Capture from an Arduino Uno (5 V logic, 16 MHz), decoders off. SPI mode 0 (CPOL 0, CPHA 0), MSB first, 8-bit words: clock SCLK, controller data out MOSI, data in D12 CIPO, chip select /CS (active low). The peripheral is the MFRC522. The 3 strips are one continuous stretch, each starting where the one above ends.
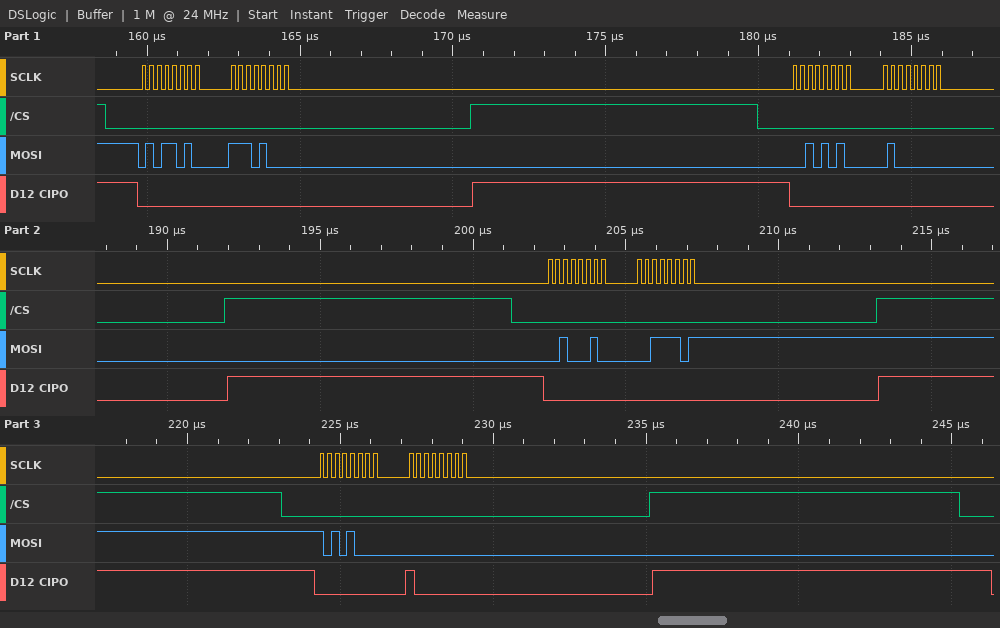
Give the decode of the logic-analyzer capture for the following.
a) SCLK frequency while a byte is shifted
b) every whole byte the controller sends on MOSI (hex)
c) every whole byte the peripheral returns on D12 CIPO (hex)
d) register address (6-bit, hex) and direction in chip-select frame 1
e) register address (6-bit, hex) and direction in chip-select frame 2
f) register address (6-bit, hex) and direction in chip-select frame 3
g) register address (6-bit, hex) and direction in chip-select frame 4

4 MHz
5A E8 2A 40 22 3D A8 00
00 00 00 00 00 00 00 80
0x2D write
0x15 write
0x11 write
0x14 read
